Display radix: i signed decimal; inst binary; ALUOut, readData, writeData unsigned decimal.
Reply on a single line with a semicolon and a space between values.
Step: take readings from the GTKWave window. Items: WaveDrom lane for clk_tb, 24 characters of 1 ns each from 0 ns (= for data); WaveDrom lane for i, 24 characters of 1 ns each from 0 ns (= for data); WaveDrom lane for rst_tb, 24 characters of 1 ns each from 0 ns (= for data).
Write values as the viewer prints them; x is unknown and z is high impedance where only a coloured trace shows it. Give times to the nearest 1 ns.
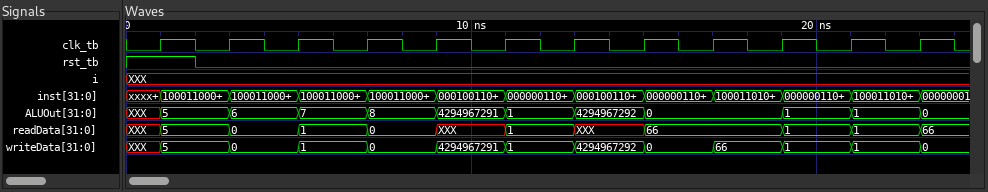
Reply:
{name: 'clk_tb', wave: '010101010101010101010101'}; {name: 'i', wave: 'x.......................'}; {name: 'rst_tb', wave: '1.0.....................'}
